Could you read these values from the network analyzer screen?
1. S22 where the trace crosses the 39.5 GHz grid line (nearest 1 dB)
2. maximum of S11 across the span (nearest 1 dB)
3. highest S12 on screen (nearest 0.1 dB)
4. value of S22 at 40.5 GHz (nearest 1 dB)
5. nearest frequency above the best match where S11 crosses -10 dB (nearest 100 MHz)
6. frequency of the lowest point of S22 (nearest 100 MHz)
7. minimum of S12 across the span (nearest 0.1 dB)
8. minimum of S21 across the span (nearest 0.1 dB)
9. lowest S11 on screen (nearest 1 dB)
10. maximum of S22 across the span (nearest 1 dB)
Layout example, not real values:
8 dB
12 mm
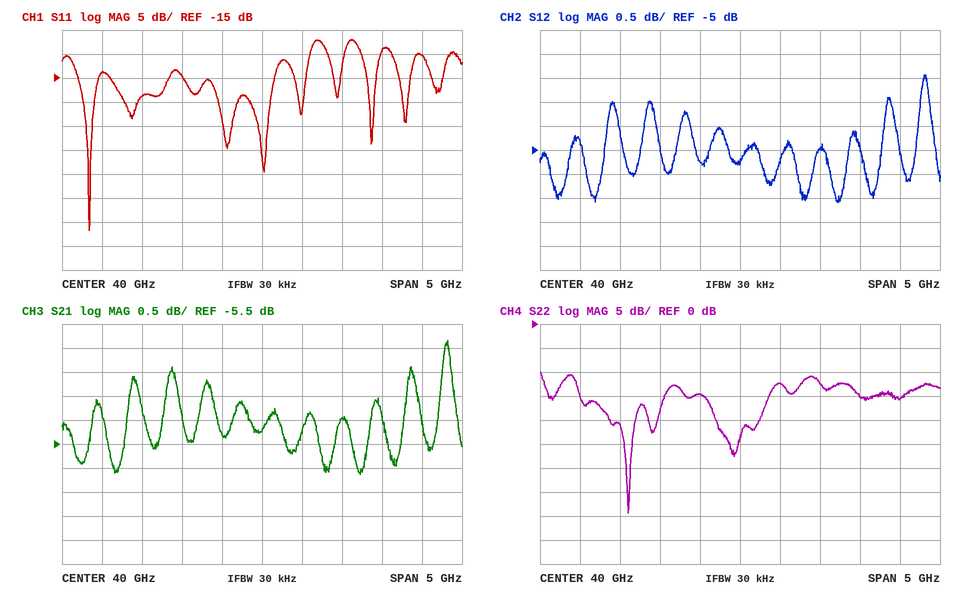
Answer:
-15 dB
-7 dB
-3.4 dB
-12 dB
40.6 GHz
38.6 GHz
-6.1 dB
-6.1 dB
-47 dB
-10 dB
